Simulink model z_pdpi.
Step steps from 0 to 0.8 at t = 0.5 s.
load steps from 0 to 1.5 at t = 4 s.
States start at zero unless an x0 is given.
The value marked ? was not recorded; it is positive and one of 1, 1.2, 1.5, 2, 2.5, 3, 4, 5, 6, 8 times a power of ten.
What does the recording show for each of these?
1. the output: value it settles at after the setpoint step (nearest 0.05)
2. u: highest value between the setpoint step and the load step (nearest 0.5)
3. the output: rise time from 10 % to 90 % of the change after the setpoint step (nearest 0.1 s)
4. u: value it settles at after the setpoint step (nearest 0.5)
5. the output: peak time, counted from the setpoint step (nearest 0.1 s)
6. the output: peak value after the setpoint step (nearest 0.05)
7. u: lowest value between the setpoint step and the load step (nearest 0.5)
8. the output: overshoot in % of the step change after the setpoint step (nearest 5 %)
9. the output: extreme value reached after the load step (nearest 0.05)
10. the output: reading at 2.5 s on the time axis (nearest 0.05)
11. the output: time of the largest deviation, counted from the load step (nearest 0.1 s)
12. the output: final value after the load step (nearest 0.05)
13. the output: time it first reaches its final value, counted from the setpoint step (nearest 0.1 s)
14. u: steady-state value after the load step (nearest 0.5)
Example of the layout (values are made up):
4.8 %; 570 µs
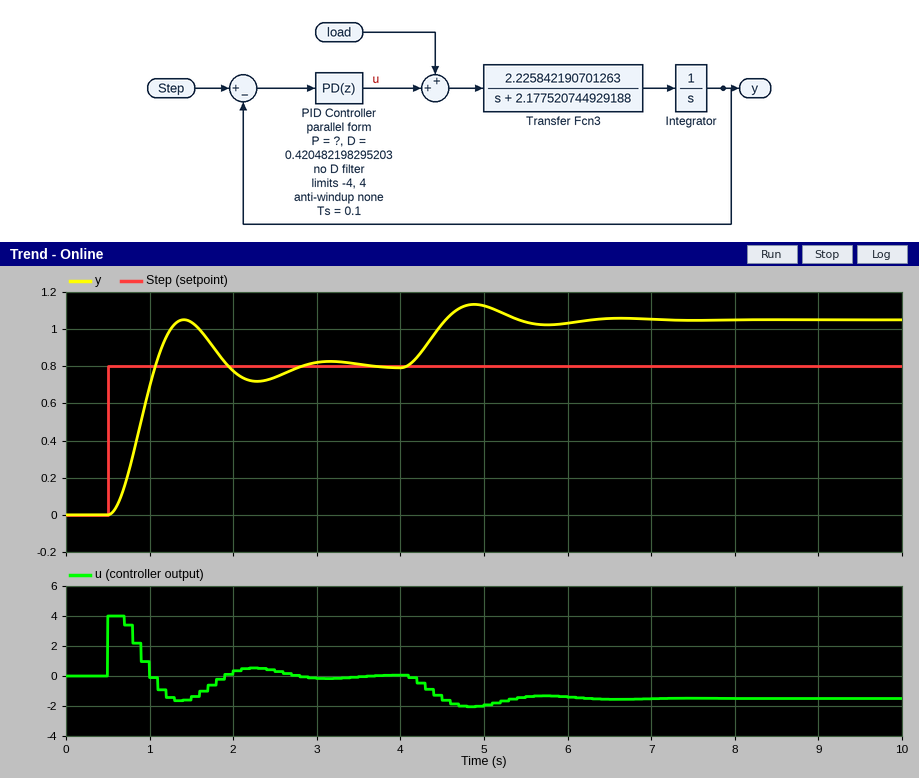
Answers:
0.80; 4.0; 0.4 s; 0.0; 0.9 s; 1.05; -1.5; 30 %; 1.15; 0.75; 0.9 s; 1.05; 0.6 s; -1.5
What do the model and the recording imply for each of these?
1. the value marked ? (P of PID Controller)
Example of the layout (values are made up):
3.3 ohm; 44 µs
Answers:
6
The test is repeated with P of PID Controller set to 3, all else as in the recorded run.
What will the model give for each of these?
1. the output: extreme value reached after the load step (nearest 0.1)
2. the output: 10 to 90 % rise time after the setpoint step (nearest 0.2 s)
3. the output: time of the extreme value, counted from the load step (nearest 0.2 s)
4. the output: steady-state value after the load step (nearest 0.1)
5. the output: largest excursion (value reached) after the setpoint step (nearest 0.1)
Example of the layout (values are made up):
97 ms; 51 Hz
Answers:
1.4; 0.6 s; 1.4 s; 1.3; 0.9
